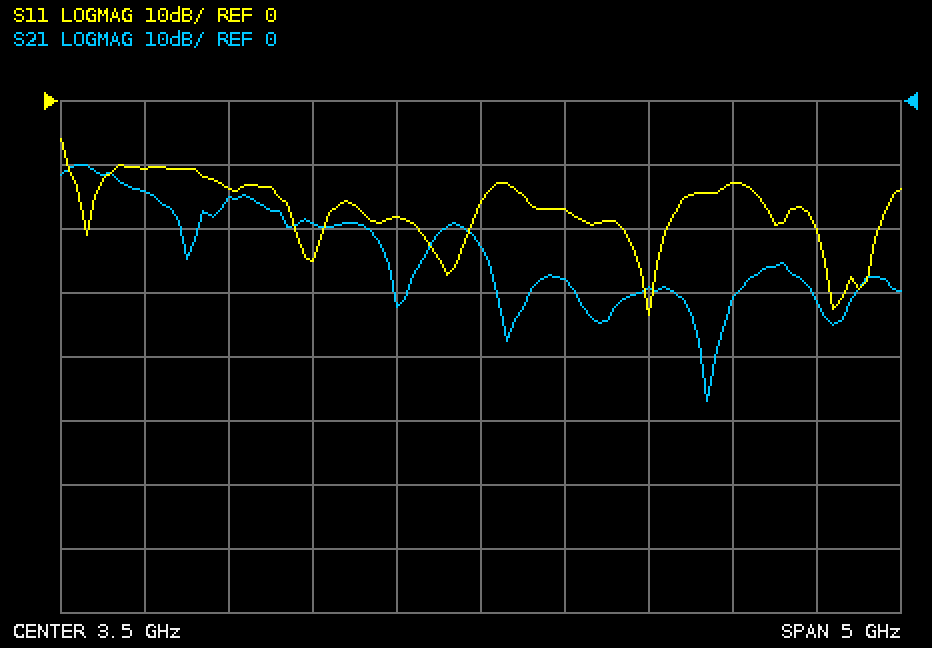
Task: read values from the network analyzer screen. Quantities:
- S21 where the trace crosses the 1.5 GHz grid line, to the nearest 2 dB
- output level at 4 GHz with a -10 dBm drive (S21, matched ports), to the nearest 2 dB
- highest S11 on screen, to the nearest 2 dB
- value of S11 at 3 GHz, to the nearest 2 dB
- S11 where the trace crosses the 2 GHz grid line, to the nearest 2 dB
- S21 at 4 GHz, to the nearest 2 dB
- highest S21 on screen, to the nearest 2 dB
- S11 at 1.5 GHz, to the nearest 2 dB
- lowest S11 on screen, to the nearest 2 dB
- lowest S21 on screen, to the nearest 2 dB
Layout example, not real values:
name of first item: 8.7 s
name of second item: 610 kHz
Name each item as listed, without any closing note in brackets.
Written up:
S21 where the trace crosses the 1.5 GHz grid line, to the nearest 2 dB: -14 dB
output level at 4 GHz with a -10 dBm drive (S21, matched ports), to the nearest 2 dB: -38 dBm
highest S11 on screen, to the nearest 2 dB: -6 dB
value of S11 at 3 GHz, to the nearest 2 dB: -18 dB
S11 where the trace crosses the 2 GHz grid line, to the nearest 2 dB: -14 dB
S21 at 4 GHz, to the nearest 2 dB: -28 dB
highest S21 on screen, to the nearest 2 dB: -10 dB
S11 at 1.5 GHz, to the nearest 2 dB: -10 dB
lowest S11 on screen, to the nearest 2 dB: -34 dB
lowest S21 on screen, to the nearest 2 dB: -46 dB
